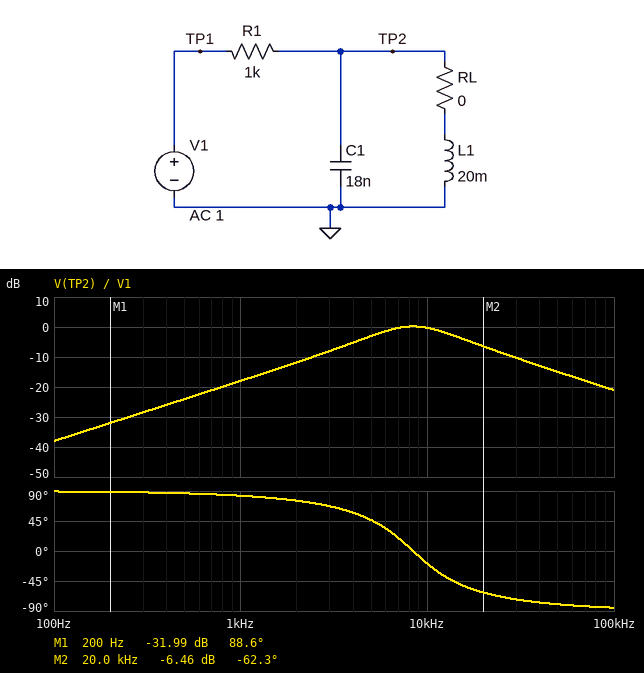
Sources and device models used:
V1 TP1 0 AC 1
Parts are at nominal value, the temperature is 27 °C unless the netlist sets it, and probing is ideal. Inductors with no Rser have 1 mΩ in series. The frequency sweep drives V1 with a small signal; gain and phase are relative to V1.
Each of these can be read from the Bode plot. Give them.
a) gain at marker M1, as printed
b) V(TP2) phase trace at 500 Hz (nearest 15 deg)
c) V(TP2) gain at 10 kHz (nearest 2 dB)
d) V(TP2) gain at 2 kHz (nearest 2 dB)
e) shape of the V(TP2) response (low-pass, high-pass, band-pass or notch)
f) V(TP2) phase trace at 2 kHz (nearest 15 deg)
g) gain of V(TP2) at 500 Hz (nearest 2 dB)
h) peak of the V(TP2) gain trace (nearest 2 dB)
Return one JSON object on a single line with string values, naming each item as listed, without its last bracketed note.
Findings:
{"gain at marker M1, as printed": "-31.99 dB", "V(TP2) phase trace at 500 Hz": "90 deg", "V(TP2) gain at 10 kHz": "0 dB", "V(TP2) gain at 2 kHz": "-12 dB", "shape of the V(TP2) response": "band-pass", "V(TP2) phase trace at 2 kHz": "75 deg", "gain of V(TP2) at 500 Hz": "-24 dB", "peak of the V(TP2) gain trace": "0 dB"}
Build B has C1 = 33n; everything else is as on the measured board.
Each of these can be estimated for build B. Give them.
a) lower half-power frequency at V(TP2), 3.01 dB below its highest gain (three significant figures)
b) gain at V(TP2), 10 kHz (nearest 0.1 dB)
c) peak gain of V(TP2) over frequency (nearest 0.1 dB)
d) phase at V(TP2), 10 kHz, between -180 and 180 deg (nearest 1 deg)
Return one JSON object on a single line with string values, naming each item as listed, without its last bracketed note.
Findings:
{"lower half-power frequency at V(TP2), 3.01 dB below its highest gain": "4.27 kHz", "gain at V(TP2), 10 kHz": "-4.1 dB", "peak gain of V(TP2) over frequency": "0.2 dB", "phase at V(TP2), 10 kHz, between -180 and 180 deg": "-53 deg"}
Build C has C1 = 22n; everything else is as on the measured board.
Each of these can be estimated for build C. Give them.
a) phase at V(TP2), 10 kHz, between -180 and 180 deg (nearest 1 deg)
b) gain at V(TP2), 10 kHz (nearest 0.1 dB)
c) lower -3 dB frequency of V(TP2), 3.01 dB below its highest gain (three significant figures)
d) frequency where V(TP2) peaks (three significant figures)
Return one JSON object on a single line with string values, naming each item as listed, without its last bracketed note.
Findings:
{"phase at V(TP2), 10 kHz, between -180 and 180 deg": "-31 deg", "gain at V(TP2), 10 kHz": "-1.1 dB", "lower -3 dB frequency of V(TP2), 3.01 dB below its highest gain": "4.84 kHz", "frequency where V(TP2) peaks": "7.59 kHz"}
